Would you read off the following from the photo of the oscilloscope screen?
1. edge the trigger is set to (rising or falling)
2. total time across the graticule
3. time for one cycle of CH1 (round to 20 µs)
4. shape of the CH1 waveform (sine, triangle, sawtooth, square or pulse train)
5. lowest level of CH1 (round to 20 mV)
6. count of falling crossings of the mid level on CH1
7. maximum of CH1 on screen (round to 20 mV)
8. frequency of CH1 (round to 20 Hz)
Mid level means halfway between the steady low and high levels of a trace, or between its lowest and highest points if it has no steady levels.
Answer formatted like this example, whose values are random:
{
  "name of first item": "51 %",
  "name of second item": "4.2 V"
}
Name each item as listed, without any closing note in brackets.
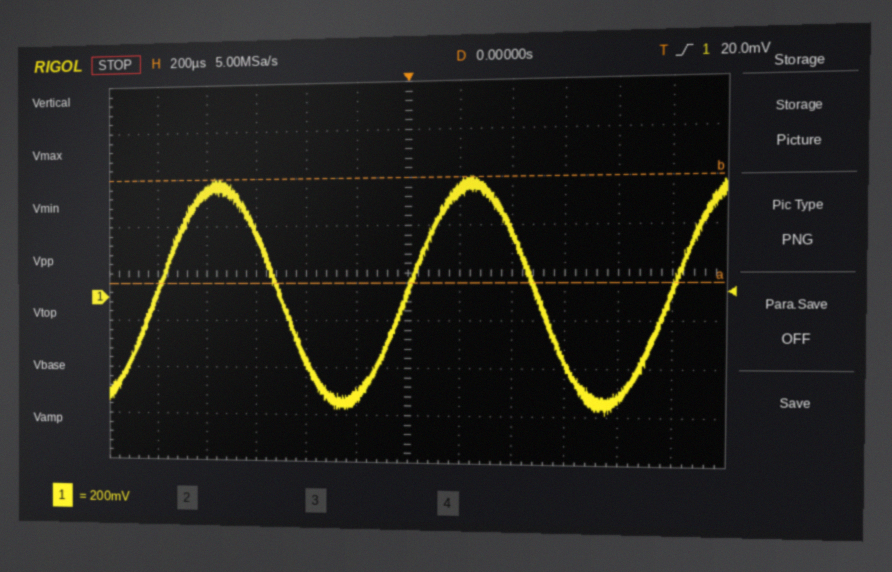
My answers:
{
  "edge the trigger is set to": "rising",
  "total time across the graticule": "2.4 ms",
  "time for one cycle of CH1": "1.00 ms",
  "shape of the CH1 waveform": "sine",
  "lowest level of CH1": "-480 mV",
  "count of falling crossings of the mid level on CH1": "2",
  "maximum of CH1 on screen": "500 mV",
  "frequency of CH1": "1.00 kHz"
}
